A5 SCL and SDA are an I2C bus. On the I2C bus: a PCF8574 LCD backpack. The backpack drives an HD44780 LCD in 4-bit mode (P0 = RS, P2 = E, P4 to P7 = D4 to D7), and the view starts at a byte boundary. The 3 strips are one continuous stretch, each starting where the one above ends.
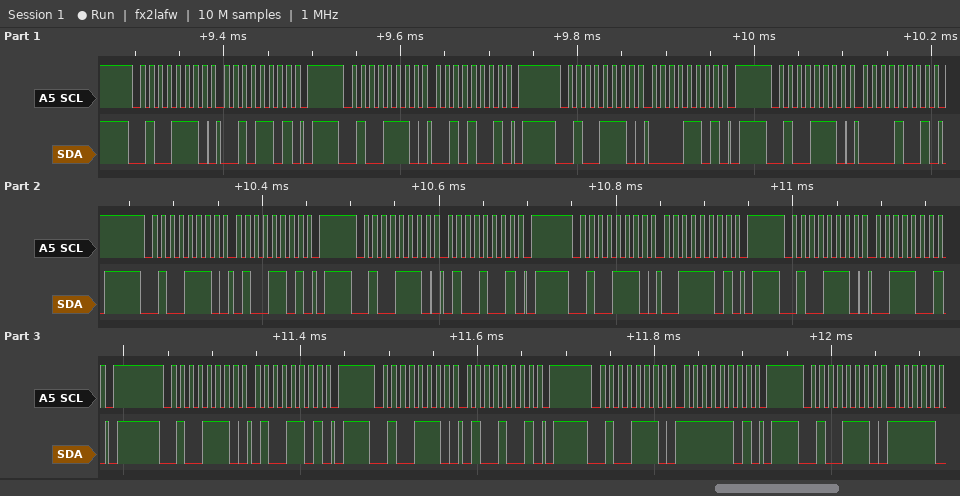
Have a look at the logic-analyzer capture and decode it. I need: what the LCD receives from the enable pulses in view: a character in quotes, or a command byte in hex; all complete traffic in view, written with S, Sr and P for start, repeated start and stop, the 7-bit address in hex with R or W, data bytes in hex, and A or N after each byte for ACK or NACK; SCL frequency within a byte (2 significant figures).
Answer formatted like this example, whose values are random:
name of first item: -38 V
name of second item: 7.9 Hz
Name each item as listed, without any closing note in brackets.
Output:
what the LCD receives from the enable pulses in view: a character in quotes, or a command byte in hex: ' ' 'C'
all complete traffic in view, written with S, Sr and P for start, repeated start and stop, the 7-bit address in hex with R or W, data bytes in hex, and A or N after each byte for ACK or NACK: S 27W A 2D A P S 27W A 29 A P S 27W A 0D A P S 27W A 09 A P S 27W A 4D A P S 27W A 49 A P S 27W A 3D A P S 27W A 39 A P S 27W A 4D A P S 27W A 49 A P S 27W A FD A P S 27W A
SCL frequency within a byte: 100 kHz
